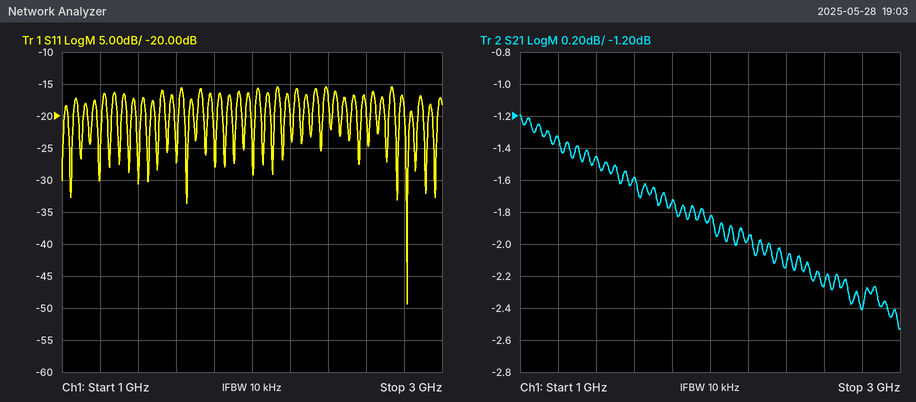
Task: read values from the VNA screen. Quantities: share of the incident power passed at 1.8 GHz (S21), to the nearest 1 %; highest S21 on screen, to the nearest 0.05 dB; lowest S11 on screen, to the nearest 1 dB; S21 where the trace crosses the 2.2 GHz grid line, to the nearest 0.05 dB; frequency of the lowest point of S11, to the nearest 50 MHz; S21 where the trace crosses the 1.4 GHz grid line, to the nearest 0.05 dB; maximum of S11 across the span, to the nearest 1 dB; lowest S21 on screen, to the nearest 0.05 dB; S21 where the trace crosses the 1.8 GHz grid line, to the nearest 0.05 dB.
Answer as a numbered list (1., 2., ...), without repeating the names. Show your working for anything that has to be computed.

1. 10^(-1.75/10) ≈ 67 %
2. -1.20 dB
3. -49 dB
4. -1.95 dB
5. 2.80 GHz
6. -1.45 dB
7. -15 dB
8. -2.55 dB
9. -1.75 dB
